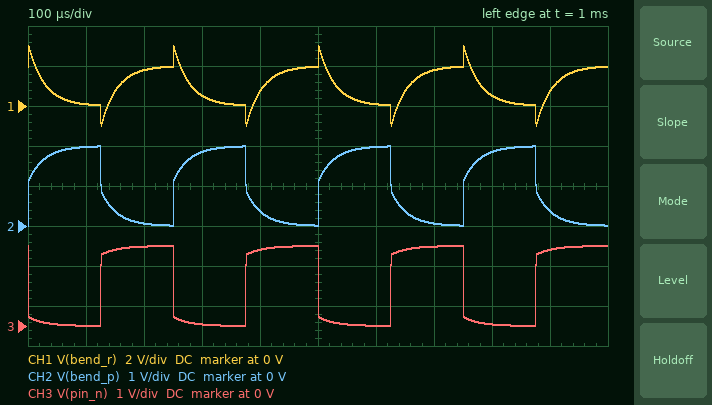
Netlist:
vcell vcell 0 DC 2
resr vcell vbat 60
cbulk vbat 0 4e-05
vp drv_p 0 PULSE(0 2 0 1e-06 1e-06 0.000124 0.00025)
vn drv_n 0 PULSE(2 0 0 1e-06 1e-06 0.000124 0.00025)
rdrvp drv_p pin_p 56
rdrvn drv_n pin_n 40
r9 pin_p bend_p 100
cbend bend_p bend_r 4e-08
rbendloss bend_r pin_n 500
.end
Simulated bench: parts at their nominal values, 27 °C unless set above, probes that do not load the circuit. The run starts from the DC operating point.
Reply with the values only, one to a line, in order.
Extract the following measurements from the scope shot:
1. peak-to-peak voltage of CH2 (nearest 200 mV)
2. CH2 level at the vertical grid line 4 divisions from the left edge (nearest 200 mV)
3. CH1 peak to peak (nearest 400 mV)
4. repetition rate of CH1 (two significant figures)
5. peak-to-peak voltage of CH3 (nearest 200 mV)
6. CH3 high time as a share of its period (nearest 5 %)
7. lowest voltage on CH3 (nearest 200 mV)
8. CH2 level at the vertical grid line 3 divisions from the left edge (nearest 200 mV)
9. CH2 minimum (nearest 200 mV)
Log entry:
2.0 V
400 mV
4.0 V
4.0 kHz
2.0 V
50 %
0 V
1.8 V
0 V
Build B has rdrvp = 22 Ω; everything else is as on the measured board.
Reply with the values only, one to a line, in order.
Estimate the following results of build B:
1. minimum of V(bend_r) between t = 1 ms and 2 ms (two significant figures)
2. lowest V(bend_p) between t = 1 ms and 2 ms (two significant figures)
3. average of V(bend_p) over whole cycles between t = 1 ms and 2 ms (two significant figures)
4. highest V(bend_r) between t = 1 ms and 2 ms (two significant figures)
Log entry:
-1.2 V
6.6 mV
1.0 V
3.2 V
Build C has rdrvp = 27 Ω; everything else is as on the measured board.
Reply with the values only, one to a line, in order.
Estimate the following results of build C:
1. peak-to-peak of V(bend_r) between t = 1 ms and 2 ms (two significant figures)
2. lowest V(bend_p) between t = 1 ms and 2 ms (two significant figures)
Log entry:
4.3 V
7.1 mV
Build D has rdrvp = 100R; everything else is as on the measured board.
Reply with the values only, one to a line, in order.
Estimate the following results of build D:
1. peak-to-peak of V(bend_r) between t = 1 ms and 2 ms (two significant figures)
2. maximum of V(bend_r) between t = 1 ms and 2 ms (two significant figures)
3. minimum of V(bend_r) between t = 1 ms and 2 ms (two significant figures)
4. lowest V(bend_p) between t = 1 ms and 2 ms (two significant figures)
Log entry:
3.7 V
2.8 V
-830 mV
16 mV
